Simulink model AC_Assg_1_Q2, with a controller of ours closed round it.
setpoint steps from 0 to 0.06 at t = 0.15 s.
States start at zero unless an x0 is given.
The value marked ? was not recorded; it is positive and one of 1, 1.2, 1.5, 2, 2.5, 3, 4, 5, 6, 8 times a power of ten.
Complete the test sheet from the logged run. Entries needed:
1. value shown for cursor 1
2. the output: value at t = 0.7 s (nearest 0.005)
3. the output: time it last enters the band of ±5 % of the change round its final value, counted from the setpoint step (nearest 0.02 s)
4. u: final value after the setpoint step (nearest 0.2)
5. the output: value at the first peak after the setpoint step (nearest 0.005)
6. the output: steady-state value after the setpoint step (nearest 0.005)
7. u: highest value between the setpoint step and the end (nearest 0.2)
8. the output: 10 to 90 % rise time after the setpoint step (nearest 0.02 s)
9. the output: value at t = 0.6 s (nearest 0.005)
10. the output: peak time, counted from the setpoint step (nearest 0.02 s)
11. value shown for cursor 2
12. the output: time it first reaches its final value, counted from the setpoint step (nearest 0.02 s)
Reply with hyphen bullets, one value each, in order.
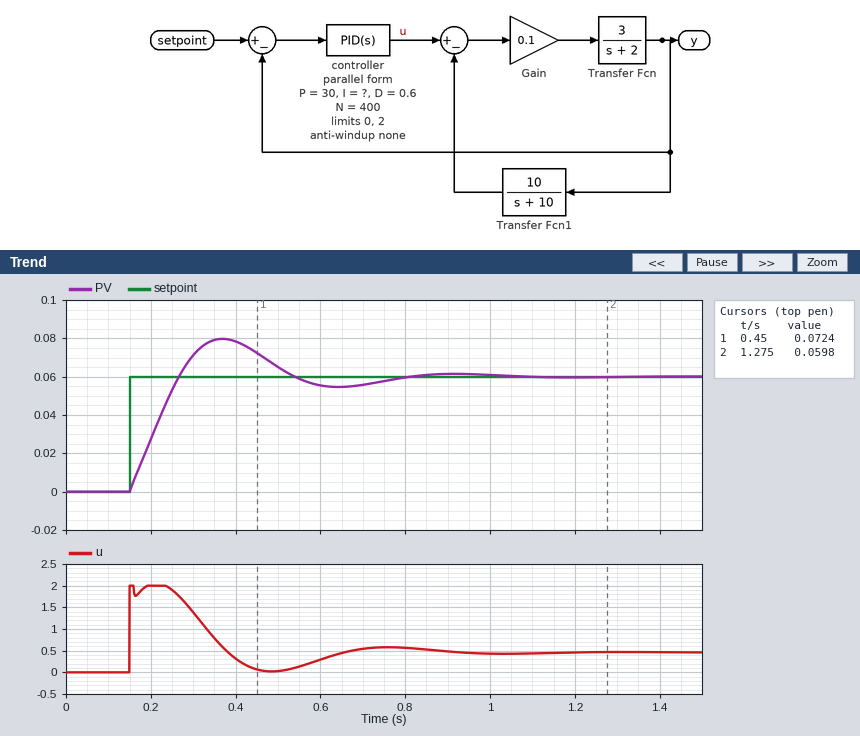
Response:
- 0.0724
- 0.055
- 0.58 s
- 0.4
- 0.080
- 0.060
- 2.0
- 0.10 s
- 0.055
- 0.22 s
- 0.0598
- 0.12 s
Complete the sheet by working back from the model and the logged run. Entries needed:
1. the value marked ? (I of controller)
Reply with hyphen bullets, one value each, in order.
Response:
- 600
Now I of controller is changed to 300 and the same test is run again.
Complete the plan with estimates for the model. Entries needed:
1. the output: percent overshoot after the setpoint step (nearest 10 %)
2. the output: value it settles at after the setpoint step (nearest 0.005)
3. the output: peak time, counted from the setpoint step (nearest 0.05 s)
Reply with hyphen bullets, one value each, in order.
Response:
- 20 %
- 0.060
- 0.30 s
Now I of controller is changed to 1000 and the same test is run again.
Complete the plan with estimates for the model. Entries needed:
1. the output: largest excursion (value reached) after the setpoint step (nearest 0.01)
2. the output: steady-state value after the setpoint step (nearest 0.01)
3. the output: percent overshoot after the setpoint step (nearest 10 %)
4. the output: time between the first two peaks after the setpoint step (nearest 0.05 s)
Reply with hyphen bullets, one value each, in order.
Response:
- 0.09
- 0.06
- 50 %
- 0.55 s
